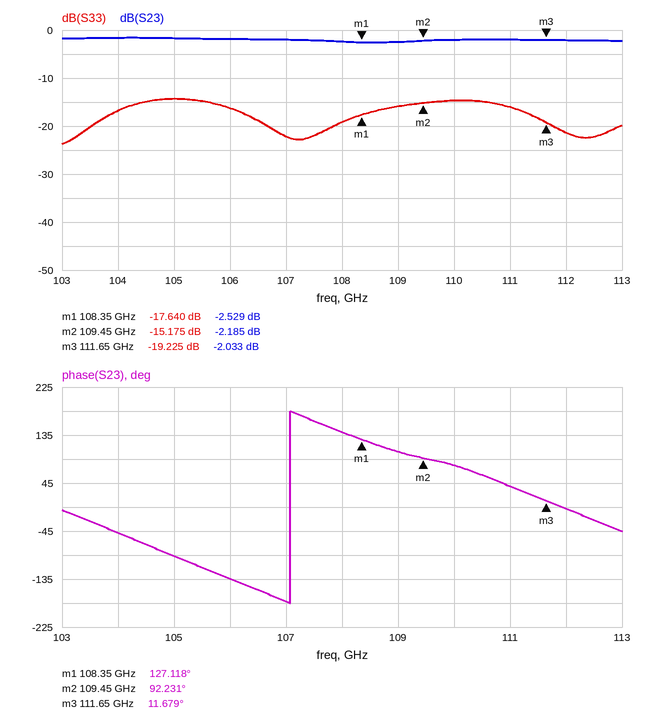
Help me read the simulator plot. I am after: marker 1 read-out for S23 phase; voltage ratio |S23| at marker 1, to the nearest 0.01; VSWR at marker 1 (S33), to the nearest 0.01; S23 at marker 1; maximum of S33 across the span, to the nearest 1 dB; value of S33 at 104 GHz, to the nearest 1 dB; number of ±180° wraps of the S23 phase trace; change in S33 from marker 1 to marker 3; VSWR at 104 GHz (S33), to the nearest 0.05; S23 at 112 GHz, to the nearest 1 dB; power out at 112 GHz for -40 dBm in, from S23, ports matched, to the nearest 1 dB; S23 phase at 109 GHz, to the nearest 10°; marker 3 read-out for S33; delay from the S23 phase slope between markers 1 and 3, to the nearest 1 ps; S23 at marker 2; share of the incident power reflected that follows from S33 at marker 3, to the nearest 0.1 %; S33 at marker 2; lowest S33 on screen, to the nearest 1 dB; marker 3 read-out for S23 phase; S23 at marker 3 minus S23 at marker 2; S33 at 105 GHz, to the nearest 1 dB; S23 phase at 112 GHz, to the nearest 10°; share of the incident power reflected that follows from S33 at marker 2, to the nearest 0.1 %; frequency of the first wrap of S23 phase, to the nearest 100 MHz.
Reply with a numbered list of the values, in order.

1. 127.118°
2. 0.75
3. 1.30
4. -2.529 dB
5. -14 dB
6. -17 dB
7. 1
8. -1.585 dB
9. 1.35
10. -2 dB
11. -42 dBm
12. 100°
13. -19.225 dB
14. 97 ps
15. -2.185 dB
16. 1.2 %
17. -15.175 dB
18. -24 dB
19. 11.679°
20. 0.152 dB
21. -14 dB
22. 0°
23. 3.0 %
24. 107.1 GHz
